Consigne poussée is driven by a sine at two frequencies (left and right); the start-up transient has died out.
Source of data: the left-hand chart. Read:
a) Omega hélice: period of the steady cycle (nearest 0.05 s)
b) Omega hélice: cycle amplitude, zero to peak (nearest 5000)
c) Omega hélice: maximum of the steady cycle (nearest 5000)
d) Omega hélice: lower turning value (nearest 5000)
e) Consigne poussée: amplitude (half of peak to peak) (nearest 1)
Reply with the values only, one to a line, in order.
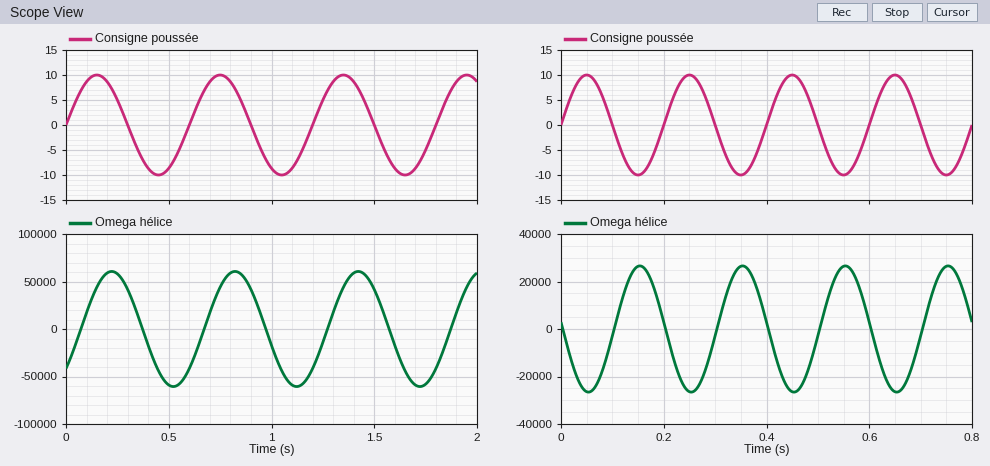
0.60 s
60000
60000
-60000
10
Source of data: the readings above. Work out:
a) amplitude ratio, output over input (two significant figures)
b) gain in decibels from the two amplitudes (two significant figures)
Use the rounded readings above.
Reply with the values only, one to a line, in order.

6000
76 dB
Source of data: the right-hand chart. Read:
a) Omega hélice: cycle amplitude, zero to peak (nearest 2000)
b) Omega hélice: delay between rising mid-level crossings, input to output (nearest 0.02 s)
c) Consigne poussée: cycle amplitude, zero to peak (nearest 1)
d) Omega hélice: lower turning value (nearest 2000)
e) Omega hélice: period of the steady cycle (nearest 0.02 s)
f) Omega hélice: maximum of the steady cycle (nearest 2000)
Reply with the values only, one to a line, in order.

26000
0.10 s
10
-26000
0.20 s
26000
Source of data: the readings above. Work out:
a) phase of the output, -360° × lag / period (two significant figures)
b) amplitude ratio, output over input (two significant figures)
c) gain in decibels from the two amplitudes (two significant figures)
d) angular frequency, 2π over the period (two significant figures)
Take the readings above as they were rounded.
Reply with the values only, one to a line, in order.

-180°
2600
68 dB
31 rad/s
